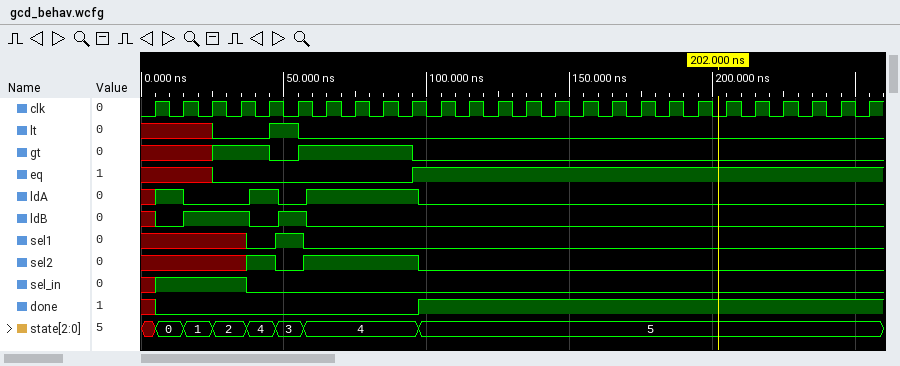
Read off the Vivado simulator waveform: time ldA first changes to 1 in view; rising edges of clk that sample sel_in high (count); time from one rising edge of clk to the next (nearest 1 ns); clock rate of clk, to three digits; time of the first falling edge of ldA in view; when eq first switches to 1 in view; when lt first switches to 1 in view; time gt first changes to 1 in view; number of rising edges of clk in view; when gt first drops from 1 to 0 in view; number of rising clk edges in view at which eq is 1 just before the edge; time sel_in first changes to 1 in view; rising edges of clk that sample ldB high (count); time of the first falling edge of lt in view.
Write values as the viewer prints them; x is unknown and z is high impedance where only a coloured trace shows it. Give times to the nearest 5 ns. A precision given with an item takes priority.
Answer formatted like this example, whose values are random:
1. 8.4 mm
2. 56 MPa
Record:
1. 5 ns
2. 3
3. 10 ns
4. 100 MHz
5. 15 ns
6. 95 ns
7. 45 ns
8. 25 ns
9. 26
10. 45 ns
11. 16
12. 5 ns
13. 3
14. 55 ns
